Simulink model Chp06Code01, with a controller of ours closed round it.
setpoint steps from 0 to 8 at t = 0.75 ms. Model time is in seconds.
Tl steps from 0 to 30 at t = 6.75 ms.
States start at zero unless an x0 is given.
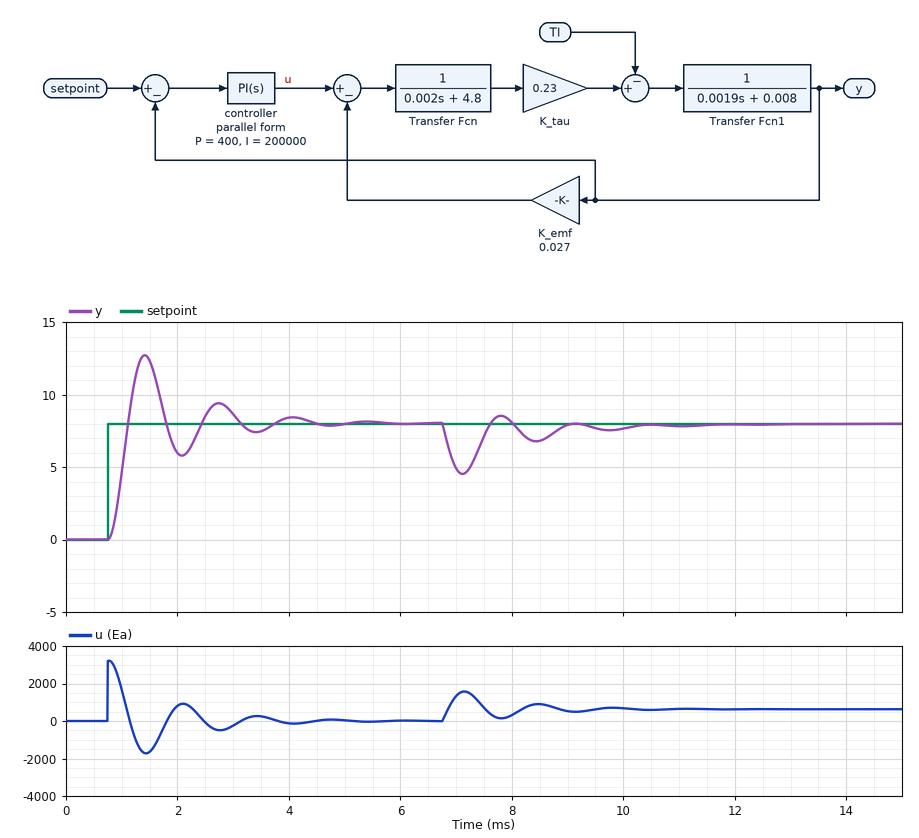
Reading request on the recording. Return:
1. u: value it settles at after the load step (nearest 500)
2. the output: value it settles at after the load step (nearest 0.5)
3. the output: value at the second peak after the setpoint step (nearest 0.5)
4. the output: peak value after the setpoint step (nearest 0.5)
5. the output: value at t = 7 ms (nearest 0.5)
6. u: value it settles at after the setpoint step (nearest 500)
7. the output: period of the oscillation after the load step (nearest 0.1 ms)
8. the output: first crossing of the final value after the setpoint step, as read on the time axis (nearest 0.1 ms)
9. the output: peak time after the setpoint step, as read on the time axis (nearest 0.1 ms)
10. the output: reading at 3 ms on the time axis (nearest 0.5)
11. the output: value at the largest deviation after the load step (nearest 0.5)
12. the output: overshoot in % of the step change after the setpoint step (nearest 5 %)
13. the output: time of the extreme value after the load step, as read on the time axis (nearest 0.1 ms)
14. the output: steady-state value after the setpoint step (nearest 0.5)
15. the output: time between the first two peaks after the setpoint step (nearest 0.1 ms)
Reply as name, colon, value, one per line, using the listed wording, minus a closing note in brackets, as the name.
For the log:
u: value it settles at after the load step: 500
the output: value it settles at after the load step: 8.0
the output: value at the second peak after the setpoint step: 9.5
the output: peak value after the setpoint step: 12.5
the output: value at t = 7 ms: 5.0
u: value it settles at after the setpoint step: 0
the output: period of the oscillation after the load step: 1.3 ms
the output: first crossing of the final value after the setpoint step, as read on the time axis: 1.1 ms
the output: peak time after the setpoint step, as read on the time axis: 1.4 ms
the output: reading at 3 ms on the time axis: 8.5
the output: value at the largest deviation after the load step: 4.5
the output: overshoot in % of the step change after the setpoint step: 60 %
the output: time of the extreme value after the load step, as read on the time axis: 7.1 ms
the output: steady-state value after the setpoint step: 8.0
the output: time between the first two peaks after the setpoint step: 1.3 ms
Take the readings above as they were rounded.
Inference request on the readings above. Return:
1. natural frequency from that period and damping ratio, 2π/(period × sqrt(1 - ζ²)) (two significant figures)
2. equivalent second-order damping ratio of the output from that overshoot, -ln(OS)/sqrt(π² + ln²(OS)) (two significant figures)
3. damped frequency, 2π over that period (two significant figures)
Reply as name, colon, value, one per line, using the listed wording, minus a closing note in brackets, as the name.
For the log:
natural frequency from that period and damping ratio, 2π/(period × sqrt(1 - ζ²)): 4.9 rad/ms
equivalent second-order damping ratio of the output from that overshoot, -ln(OS)/sqrt(π² + ln²(OS)): 0.16
damped frequency, 2π over that period: 4.8 rad/ms
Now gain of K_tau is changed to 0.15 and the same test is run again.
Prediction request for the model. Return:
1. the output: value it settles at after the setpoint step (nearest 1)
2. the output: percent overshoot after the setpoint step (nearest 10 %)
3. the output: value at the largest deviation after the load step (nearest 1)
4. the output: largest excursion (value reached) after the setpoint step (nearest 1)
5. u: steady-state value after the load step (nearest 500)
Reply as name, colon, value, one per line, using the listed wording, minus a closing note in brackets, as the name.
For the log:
the output: value it settles at after the setpoint step: 8
the output: percent overshoot after the setpoint step: 50 %
the output: value at the largest deviation after the load step: 4
the output: largest excursion (value reached) after the setpoint step: 12
u: steady-state value after the load step: 1000
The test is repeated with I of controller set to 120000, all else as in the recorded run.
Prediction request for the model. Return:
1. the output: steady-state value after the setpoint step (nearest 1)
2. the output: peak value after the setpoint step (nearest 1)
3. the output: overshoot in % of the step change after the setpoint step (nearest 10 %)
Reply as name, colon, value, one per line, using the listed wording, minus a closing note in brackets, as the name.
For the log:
the output: steady-state value after the setpoint step: 8
the output: peak value after the setpoint step: 12
the output: overshoot in % of the step change after the setpoint step: 50 %
